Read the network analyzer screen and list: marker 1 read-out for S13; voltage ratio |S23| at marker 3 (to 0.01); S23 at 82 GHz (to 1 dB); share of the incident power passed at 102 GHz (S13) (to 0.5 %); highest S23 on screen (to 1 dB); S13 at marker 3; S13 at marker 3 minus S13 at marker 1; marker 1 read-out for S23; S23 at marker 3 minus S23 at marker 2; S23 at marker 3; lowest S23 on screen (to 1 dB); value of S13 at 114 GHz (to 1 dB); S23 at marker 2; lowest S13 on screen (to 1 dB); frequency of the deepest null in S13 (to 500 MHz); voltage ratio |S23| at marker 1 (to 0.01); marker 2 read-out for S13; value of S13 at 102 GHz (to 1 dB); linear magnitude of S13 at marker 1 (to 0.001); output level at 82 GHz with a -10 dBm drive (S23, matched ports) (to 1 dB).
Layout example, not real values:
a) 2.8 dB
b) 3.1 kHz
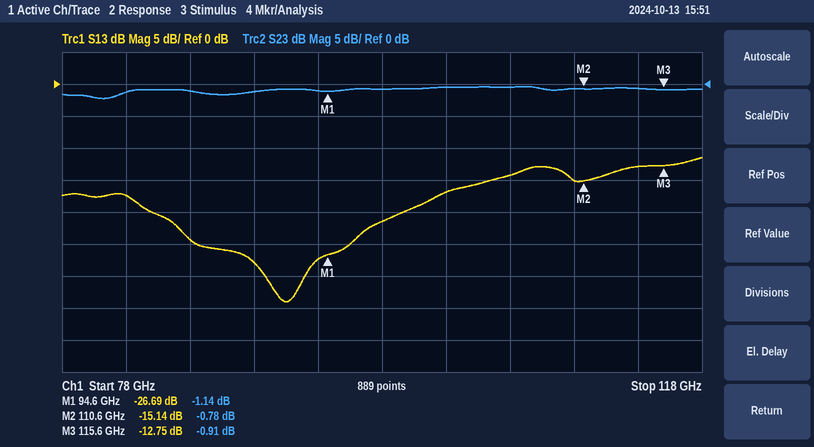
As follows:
a) -26.69 dB
b) 0.90
c) -1 dB
d) 2.0 %
e) 0 dB
f) -12.75 dB
g) 13.94 dB
h) -1.14 dB
i) -0.13 dB
j) -0.91 dB
k) -2 dB
l) -13 dB
m) -0.78 dB
n) -34 dB
o) 92.0 GHz
p) 0.88
q) -15.14 dB
r) -17 dB
s) 0.046
t) -11 dBm
